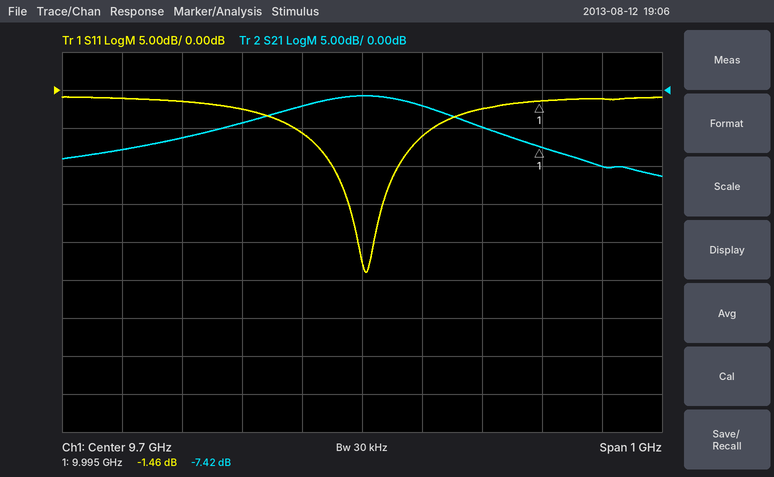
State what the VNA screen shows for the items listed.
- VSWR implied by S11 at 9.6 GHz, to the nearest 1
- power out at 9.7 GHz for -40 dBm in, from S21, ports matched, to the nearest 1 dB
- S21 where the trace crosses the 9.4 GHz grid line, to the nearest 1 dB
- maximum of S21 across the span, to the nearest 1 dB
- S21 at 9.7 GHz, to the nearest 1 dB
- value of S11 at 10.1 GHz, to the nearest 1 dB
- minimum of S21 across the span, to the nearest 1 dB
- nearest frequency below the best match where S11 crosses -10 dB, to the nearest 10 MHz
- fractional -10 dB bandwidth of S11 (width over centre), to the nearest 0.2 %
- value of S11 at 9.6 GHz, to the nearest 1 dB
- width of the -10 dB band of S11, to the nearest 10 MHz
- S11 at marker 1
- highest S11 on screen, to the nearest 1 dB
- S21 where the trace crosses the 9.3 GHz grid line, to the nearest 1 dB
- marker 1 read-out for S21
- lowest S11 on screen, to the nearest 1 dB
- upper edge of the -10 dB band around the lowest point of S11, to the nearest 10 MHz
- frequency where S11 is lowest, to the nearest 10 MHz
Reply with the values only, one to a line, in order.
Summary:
3
-41 dBm
-6 dB
-1 dB
-1 dB
-1 dB
-11 dB
9.65 GHz
1.2 %
-6 dB
110 MHz
-1.46 dB
-1 dB
-8 dB
-7.42 dB
-24 dB
9.76 GHz
9.71 GHz
